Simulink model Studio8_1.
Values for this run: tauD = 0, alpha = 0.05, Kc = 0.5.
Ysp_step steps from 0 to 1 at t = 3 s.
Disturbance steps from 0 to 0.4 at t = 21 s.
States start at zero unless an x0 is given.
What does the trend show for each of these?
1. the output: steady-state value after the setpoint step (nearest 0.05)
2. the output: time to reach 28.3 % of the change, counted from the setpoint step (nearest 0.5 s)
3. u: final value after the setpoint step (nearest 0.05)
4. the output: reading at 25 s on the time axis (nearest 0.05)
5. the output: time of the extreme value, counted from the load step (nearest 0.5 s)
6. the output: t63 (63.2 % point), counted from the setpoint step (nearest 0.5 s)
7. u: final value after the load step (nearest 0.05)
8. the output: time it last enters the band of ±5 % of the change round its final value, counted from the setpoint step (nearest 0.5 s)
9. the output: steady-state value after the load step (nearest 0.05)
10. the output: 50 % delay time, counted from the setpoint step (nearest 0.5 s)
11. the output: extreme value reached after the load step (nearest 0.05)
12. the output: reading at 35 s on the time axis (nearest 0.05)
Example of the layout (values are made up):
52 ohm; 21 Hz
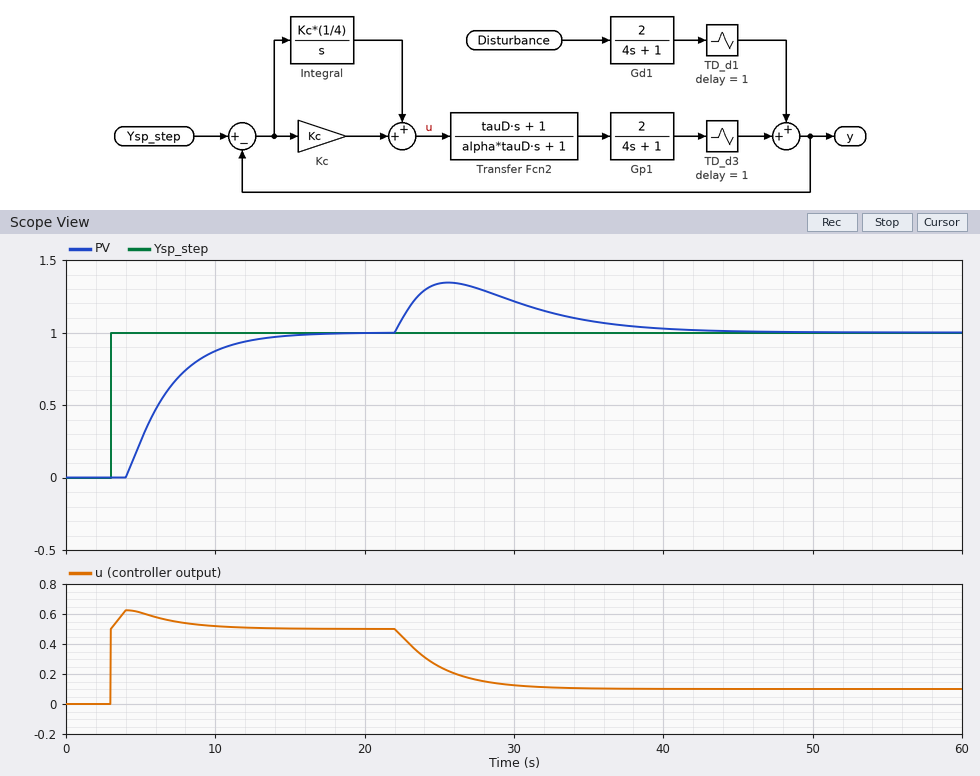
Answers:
1.00; 2.0 s; 0.50; 1.35; 4.5 s; 4.0 s; 0.10; 9.5 s; 1.00; 3.0 s; 1.35; 1.10
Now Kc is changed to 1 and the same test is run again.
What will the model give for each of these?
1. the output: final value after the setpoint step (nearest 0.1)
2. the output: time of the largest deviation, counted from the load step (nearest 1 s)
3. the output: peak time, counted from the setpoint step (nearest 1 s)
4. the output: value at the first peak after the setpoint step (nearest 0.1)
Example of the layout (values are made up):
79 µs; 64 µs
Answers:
1.0; 3 s; 5 s; 1.0
